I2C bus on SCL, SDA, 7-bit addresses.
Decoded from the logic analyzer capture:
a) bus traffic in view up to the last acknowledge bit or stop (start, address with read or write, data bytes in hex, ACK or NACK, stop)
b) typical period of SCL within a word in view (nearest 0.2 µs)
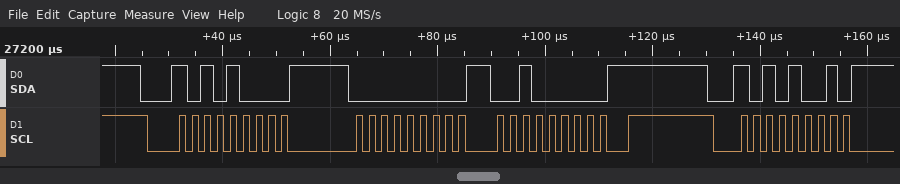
start, address 54 write ACK, 00 ACK, 20 ACK, repeated start, address 54 read ACK
2.4 µs
